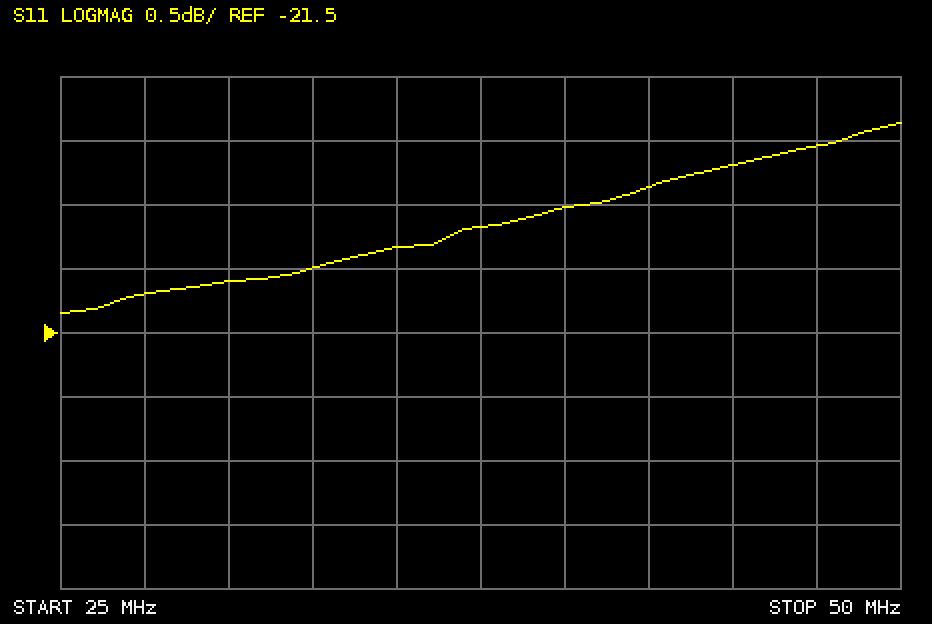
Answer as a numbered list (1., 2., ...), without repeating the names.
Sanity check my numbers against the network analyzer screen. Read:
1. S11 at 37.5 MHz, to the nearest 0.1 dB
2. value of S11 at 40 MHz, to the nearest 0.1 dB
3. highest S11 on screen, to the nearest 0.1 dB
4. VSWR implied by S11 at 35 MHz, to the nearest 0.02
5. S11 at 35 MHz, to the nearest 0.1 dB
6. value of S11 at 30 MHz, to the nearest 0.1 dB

1. -20.7 dB
2. -20.5 dB
3. -19.9 dB
4. 1.20
5. -20.8 dB
6. -21.1 dB
